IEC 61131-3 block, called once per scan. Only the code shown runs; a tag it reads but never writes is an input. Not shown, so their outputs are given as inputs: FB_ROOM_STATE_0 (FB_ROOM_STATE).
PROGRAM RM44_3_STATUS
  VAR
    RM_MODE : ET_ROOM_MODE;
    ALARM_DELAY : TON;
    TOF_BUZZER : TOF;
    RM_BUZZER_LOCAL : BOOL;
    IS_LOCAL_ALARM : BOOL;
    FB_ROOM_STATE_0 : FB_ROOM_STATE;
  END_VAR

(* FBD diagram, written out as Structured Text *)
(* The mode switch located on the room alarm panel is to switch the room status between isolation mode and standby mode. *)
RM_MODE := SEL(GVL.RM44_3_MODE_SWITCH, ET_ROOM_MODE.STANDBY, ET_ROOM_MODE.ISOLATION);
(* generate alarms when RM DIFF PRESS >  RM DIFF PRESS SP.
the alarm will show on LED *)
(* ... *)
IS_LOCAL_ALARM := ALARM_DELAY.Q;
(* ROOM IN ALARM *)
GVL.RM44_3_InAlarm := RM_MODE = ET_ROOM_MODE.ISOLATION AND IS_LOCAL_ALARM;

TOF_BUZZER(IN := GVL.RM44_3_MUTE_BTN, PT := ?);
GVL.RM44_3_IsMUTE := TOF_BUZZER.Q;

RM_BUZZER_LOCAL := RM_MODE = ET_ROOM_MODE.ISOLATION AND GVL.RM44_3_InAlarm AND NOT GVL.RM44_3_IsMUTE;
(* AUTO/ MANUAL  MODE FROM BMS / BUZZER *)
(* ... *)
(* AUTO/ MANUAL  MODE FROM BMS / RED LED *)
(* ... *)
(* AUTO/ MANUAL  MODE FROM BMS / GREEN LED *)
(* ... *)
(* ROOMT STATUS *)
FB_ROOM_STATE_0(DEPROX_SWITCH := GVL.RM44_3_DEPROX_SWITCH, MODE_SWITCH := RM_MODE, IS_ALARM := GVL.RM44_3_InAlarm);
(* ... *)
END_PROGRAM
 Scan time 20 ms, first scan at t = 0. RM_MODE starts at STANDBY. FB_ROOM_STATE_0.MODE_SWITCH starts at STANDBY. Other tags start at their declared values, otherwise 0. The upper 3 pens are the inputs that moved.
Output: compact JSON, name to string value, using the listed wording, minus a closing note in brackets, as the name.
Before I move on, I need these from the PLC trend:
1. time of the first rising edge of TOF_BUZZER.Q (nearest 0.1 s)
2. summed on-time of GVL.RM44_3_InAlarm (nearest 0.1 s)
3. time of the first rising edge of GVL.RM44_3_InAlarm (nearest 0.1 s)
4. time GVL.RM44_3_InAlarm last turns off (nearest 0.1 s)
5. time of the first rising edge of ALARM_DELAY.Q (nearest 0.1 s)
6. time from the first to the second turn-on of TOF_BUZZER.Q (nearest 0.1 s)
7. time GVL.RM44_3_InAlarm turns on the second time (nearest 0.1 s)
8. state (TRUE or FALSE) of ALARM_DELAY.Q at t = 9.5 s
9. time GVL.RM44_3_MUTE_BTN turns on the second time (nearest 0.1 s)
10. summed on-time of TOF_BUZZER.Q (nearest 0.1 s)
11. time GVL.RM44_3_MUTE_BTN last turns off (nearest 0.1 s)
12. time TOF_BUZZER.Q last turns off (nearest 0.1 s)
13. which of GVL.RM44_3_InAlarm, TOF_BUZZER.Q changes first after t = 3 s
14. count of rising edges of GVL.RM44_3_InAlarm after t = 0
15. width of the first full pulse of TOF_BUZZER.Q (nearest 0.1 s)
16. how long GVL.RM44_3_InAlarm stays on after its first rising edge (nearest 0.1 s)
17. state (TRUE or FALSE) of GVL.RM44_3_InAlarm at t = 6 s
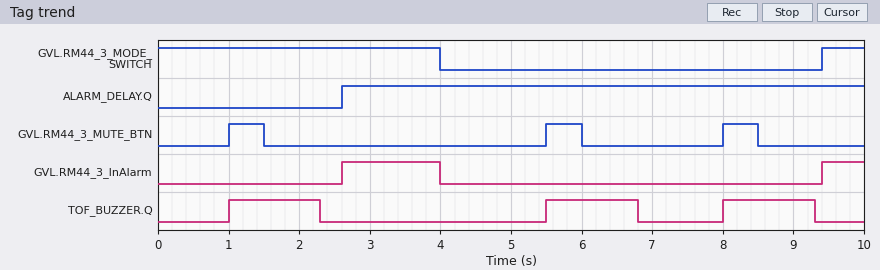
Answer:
{"time of the first rising edge of TOF_BUZZER.Q": "1.0 s", "summed on-time of GVL.RM44_3_InAlarm": "2.0 s", "time of the first rising edge of GVL.RM44_3_InAlarm": "2.6 s", "time GVL.RM44_3_InAlarm last turns off": "4.0 s", "time of the first rising edge of ALARM_DELAY.Q": "2.6 s", "time from the first to the second turn-on of TOF_BUZZER.Q": "4.5 s", "time GVL.RM44_3_InAlarm turns on the second time": "9.4 s", "state (TRUE or FALSE) of ALARM_DELAY.Q at t = 9.5 s": "TRUE", "time GVL.RM44_3_MUTE_BTN turns on the second time": "5.5 s", "summed on-time of TOF_BUZZER.Q": "3.9 s", "time GVL.RM44_3_MUTE_BTN last turns off": "8.5 s", "time TOF_BUZZER.Q last turns off": "9.3 s", "which of GVL.RM44_3_InAlarm, TOF_BUZZER.Q changes first after t = 3 s": "GVL.RM44_3_InAlarm", "count of rising edges of GVL.RM44_3_InAlarm after t = 0": "2", "width of the first full pulse of TOF_BUZZER.Q": "1.3 s", "how long GVL.RM44_3_InAlarm stays on after its first rising edge": "1.4 s", "state (TRUE or FALSE) of GVL.RM44_3_InAlarm at t = 6 s": "FALSE"}
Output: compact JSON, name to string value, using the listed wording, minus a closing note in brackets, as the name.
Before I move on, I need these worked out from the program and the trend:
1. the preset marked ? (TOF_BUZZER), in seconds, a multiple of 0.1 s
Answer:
{"the preset marked ? (TOF_BUZZER), in seconds, a multiple of 0.1 s": "0.8 s"}
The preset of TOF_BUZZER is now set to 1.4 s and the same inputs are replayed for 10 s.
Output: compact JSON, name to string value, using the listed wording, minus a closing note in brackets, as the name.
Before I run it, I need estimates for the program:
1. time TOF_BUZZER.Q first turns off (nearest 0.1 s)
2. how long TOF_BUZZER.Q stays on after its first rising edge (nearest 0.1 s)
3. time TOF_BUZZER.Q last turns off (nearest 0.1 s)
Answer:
{"time TOF_BUZZER.Q first turns off": "2.9 s", "how long TOF_BUZZER.Q stays on after its first rising edge": "1.9 s", "time TOF_BUZZER.Q last turns off": "9.9 s"}
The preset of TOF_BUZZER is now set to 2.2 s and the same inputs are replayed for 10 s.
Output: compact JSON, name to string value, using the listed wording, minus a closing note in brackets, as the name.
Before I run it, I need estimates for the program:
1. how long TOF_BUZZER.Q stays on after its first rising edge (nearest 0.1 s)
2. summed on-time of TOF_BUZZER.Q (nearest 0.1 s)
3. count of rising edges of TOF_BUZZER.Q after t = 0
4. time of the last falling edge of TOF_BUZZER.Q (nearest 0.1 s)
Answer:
{"how long TOF_BUZZER.Q stays on after its first rising edge": "2.7 s", "summed on-time of TOF_BUZZER.Q": "7.2 s", "count of rising edges of TOF_BUZZER.Q after t = 0": "2", "time of the last falling edge of TOF_BUZZER.Q": "3.7 s"}
